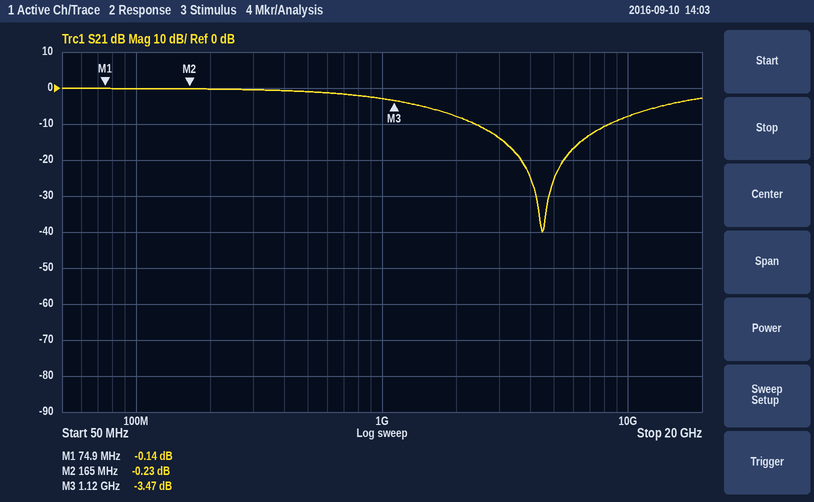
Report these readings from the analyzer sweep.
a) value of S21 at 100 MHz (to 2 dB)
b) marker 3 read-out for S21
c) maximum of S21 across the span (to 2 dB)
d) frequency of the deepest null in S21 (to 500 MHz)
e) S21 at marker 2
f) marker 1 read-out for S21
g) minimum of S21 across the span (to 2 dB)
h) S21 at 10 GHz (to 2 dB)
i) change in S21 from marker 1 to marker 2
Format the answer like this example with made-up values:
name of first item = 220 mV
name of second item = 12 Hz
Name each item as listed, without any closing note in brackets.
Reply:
value of S21 at 100 MHz = 0 dB
marker 3 read-out for S21 = -3.47 dB
maximum of S21 across the span = 0 dB
frequency of the deepest null in S21 = 4.5 GHz
S21 at marker 2 = -0.23 dB
marker 1 read-out for S21 = -0.14 dB
minimum of S21 across the span = -40 dB
S21 at 10 GHz = -8 dB
change in S21 from marker 1 to marker 2 = -0.09 dB
